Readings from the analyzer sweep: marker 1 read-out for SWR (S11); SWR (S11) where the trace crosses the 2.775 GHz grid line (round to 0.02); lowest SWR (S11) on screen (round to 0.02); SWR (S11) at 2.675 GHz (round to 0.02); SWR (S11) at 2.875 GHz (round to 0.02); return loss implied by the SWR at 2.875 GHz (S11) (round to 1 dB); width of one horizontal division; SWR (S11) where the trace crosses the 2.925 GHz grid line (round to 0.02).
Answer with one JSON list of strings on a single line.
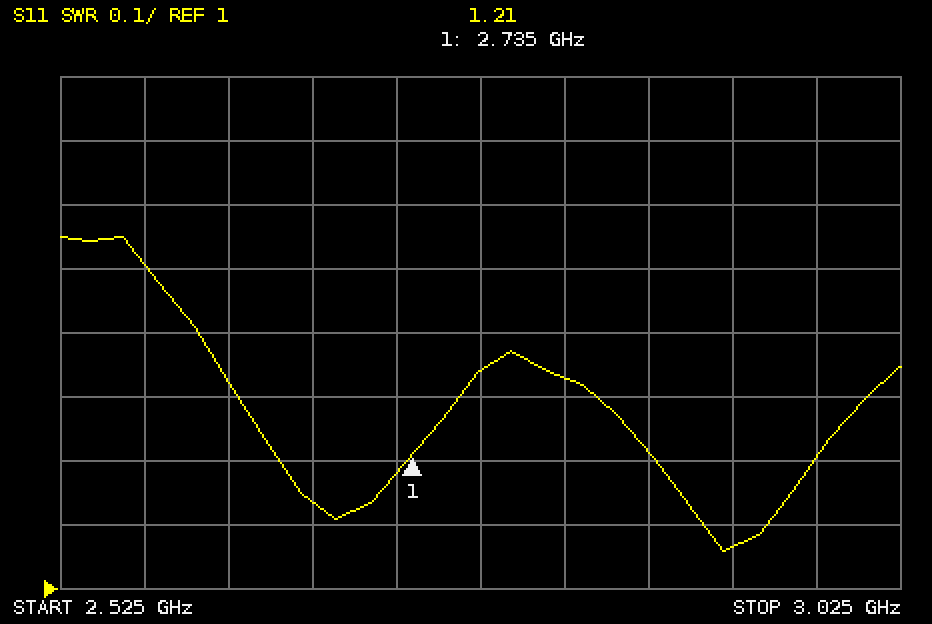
["1.21", "1.34", "1.06", "1.14", "1.22", "20 dB", "50 MHz", "1.06"]
